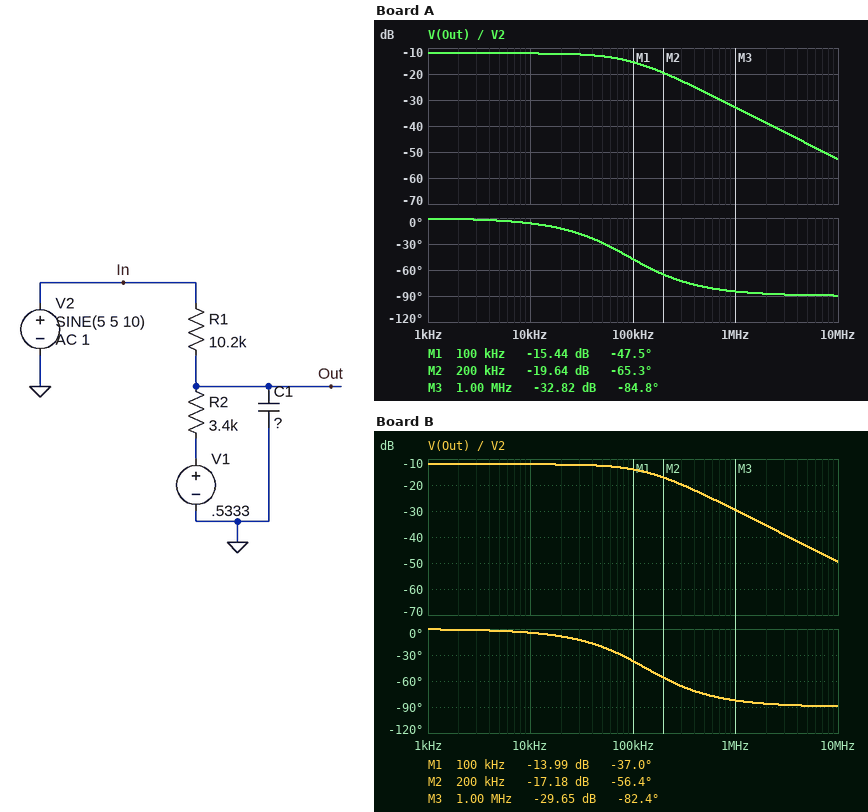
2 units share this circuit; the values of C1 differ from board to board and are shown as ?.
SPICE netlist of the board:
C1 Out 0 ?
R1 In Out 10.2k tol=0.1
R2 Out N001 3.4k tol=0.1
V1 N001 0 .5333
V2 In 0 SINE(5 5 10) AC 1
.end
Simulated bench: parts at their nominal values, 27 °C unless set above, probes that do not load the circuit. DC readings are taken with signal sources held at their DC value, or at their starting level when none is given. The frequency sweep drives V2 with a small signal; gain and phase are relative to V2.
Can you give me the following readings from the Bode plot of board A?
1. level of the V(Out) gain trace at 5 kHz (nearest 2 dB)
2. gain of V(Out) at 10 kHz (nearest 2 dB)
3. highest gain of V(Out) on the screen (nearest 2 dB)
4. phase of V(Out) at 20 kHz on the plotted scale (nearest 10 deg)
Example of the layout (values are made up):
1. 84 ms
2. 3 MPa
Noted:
1. -12 dB
2. -12 dB
3. -12 dB
4. -10 deg
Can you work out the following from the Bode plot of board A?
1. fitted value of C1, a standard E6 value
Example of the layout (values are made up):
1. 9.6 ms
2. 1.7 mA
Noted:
1. 680 pF
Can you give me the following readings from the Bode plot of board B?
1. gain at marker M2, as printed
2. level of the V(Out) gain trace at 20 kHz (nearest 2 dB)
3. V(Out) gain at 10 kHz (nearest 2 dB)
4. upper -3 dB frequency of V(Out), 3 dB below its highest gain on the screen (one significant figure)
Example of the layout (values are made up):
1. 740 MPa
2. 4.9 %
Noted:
1. -17.18 dB
2. -12 dB
3. -12 dB
4. 100 kHz
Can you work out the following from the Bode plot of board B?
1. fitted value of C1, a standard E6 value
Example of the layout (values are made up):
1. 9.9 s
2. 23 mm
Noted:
1. 470 pF
